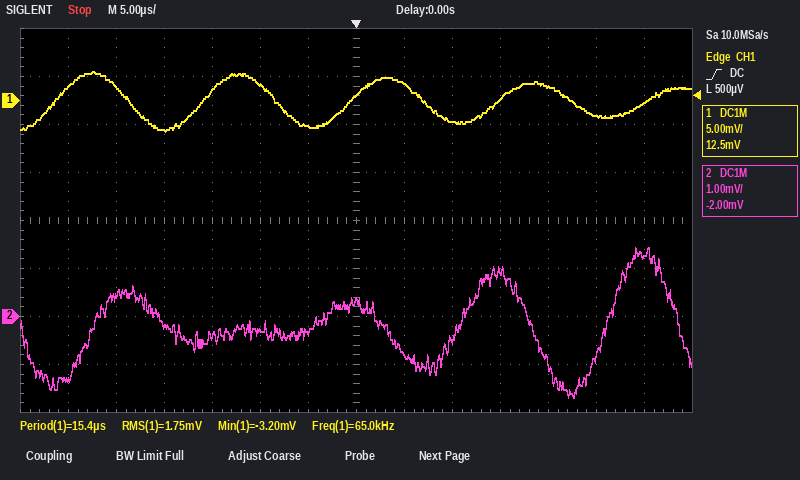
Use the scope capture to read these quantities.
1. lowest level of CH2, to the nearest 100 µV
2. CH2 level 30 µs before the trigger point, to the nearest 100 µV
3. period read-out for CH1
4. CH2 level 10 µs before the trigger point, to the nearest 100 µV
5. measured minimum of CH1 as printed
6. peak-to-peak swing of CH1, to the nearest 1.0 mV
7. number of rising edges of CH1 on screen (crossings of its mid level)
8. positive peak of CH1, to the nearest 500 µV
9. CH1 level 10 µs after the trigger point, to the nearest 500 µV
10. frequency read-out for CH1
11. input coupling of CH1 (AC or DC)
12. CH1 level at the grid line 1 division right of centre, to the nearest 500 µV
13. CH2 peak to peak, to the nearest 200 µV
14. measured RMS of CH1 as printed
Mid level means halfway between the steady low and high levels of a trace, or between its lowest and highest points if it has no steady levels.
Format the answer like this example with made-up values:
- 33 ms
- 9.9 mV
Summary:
- -1.7 mV
- -1.3 mV
- 15.4 µs
- -300 µV
- -3.20 mV
- 6.0 mV
- 5
- 3.0 mV
- -2.0 mV
- 65.0 kHz
- DC
- 2.0 mV
- 3.2 mV
- 1.75 mV
